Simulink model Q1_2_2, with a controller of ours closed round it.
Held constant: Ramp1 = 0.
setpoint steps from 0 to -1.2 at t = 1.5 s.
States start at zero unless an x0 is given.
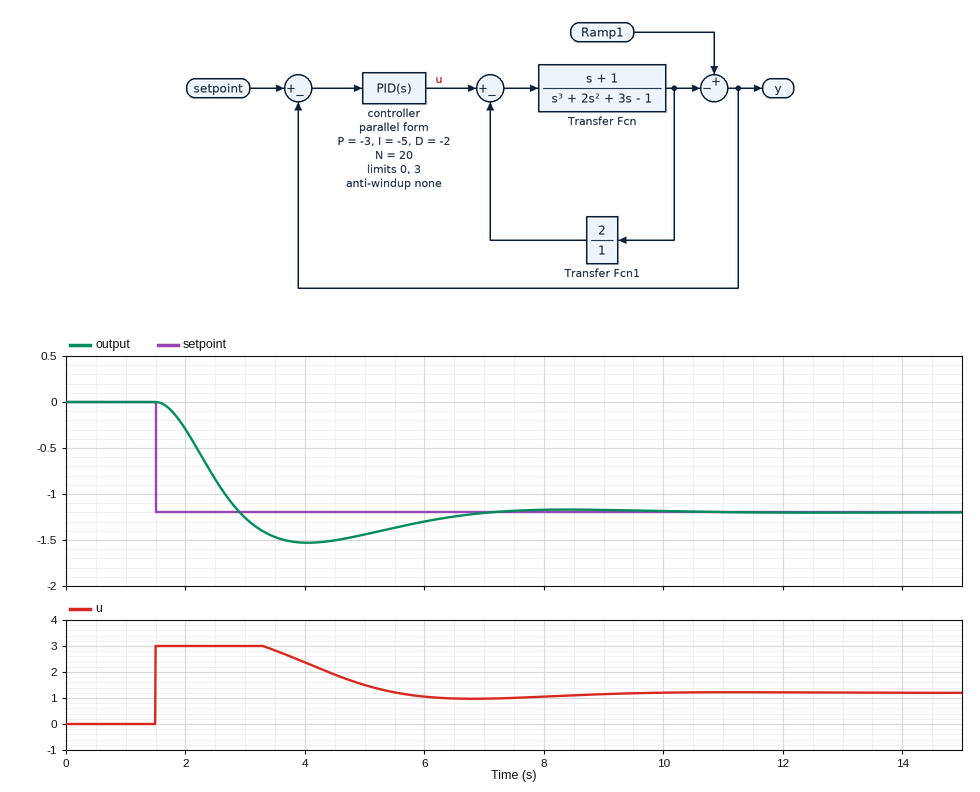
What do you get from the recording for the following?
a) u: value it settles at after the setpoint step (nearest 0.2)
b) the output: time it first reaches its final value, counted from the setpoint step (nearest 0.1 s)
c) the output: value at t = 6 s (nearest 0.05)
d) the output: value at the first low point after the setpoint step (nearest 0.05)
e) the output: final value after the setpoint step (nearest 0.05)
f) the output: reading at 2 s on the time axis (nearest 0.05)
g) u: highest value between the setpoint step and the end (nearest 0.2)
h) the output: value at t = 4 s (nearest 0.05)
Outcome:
1.2
1.4 s
-1.30
-1.55
-1.20
-0.30
3.0
-1.55
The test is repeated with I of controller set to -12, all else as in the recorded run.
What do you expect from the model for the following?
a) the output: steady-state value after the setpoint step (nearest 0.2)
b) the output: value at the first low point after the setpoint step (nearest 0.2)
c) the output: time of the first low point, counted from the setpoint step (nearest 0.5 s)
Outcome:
-1.2
-1.8
3.5 s
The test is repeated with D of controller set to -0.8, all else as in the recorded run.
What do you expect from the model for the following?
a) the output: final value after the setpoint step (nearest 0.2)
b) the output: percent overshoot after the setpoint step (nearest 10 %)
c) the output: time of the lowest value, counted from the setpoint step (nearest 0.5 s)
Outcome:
-1.2
30 %
2.5 s
